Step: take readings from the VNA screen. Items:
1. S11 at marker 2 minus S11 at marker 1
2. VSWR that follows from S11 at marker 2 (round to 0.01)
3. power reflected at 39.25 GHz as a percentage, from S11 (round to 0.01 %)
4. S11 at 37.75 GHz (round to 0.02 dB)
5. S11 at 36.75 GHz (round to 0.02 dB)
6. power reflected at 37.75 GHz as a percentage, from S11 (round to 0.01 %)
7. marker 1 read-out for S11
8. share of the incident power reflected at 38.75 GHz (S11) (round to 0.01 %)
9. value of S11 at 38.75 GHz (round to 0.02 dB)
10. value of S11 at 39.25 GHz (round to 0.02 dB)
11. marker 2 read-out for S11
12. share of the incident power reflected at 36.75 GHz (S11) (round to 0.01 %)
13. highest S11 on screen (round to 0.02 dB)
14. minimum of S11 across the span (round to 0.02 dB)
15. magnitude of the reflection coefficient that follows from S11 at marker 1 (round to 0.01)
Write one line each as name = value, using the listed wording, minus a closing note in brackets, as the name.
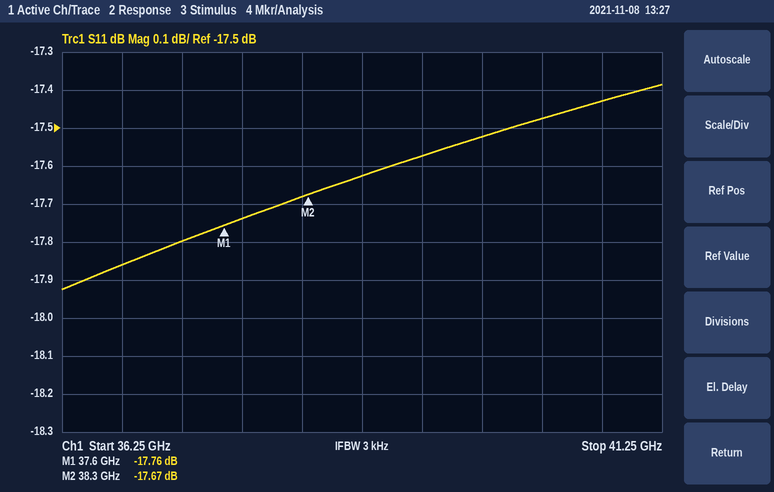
S11 at marker 2 minus S11 at marker 1 = 0.09 dB
VSWR that follows from S11 at marker 2 = 1.30
power reflected at 39.25 GHz as a percentage, from S11 = 1.75 %
S11 at 37.75 GHz = -17.74 dB
S11 at 36.75 GHz = -17.86 dB
power reflected at 37.75 GHz as a percentage, from S11 = 1.68 %
marker 1 read-out for S11 = -17.76 dB
share of the incident power reflected at 38.75 GHz (S11) = 1.73 %
value of S11 at 38.75 GHz = -17.62 dB
value of S11 at 39.25 GHz = -17.58 dB
marker 2 read-out for S11 = -17.67 dB
share of the incident power reflected at 36.75 GHz (S11) = 1.64 %
highest S11 on screen = -17.38 dB
minimum of S11 across the span = -17.92 dB
magnitude of the reflection coefficient that follows from S11 at marker 1 = 0.13
